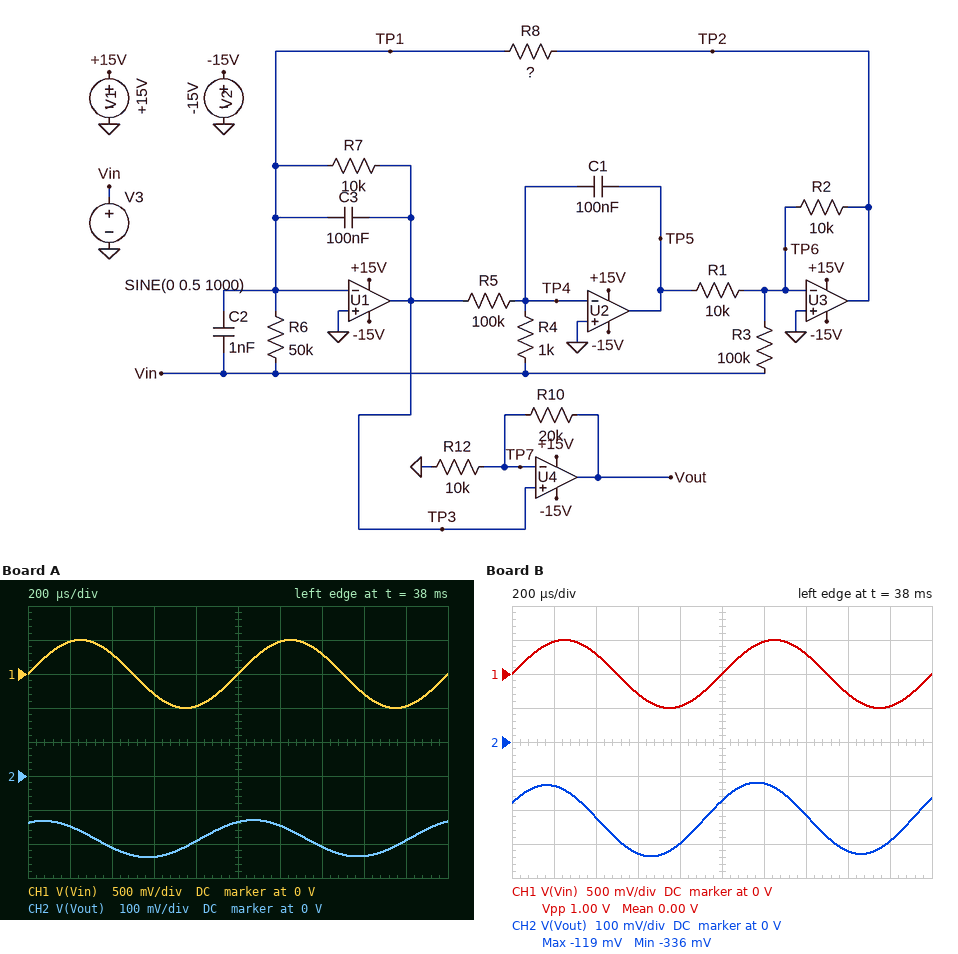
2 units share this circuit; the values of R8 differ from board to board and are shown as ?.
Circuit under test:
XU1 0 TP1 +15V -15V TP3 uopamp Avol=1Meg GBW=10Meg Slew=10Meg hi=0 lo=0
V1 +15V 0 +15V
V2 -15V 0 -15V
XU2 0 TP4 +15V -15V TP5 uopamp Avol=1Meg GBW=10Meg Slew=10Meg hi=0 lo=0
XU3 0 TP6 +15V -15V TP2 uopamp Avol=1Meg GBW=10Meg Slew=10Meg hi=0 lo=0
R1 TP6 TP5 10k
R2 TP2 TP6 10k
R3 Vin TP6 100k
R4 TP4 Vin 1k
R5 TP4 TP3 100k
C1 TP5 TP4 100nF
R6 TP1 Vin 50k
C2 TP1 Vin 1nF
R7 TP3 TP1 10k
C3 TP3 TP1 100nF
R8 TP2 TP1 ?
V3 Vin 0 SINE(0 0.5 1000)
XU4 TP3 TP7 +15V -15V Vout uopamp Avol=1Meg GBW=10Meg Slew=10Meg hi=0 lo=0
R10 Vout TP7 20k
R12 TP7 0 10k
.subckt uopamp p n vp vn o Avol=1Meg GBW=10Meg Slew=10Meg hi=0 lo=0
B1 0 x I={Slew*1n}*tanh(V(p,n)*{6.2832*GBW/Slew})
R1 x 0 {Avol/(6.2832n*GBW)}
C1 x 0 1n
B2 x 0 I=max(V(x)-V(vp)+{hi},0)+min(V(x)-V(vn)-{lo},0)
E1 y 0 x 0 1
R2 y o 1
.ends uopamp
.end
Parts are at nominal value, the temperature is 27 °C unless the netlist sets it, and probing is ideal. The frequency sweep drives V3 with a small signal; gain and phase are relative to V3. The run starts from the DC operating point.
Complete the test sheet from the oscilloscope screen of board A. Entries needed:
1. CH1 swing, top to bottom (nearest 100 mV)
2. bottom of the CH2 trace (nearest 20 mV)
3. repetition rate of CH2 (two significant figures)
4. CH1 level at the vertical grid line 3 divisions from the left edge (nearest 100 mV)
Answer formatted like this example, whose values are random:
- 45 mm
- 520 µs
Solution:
- 1.0 V
- -240 mV
- 1.0 kHz
- -300 mV
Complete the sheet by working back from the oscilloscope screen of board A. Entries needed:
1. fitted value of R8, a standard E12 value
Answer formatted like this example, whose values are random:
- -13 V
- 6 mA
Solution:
- 82 kΩ
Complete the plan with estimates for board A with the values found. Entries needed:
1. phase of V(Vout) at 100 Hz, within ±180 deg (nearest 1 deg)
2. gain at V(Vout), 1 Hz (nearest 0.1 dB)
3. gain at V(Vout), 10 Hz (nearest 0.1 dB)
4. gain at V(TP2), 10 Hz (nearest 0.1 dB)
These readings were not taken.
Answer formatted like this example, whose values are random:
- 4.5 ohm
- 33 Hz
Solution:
- 64 deg
- 48.5 dB
- 35.2 dB
- 44.0 dB
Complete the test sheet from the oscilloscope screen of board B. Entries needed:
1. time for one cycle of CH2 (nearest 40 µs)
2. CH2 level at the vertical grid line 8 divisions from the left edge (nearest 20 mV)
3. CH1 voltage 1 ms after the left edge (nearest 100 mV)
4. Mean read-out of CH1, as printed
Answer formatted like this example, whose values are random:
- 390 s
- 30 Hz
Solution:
- 1.00 ms
- -320 mV
- 0 V
- 0.00 V
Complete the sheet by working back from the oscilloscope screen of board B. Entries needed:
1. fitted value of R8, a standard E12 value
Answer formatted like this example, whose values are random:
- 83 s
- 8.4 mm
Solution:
- 33 kΩ
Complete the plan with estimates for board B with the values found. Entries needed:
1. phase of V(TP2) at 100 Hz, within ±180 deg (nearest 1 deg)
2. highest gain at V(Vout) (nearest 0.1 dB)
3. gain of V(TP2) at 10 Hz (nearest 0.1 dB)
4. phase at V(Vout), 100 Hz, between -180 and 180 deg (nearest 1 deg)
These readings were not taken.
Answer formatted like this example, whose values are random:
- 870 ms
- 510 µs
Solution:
- -88 deg
- 49.5 dB
- 43.3 dB
- 62 deg
